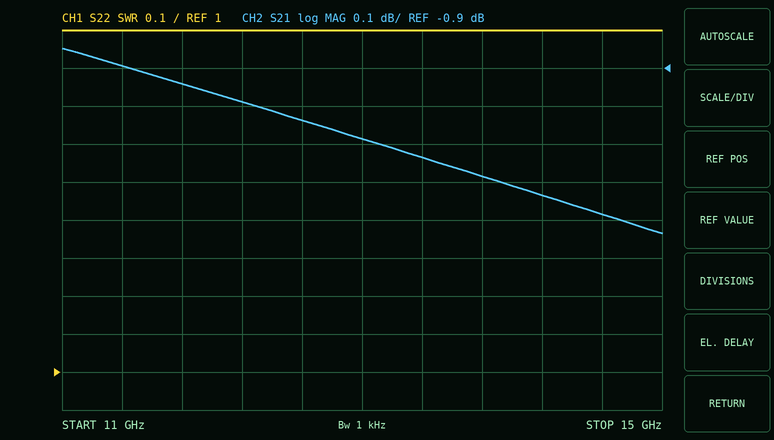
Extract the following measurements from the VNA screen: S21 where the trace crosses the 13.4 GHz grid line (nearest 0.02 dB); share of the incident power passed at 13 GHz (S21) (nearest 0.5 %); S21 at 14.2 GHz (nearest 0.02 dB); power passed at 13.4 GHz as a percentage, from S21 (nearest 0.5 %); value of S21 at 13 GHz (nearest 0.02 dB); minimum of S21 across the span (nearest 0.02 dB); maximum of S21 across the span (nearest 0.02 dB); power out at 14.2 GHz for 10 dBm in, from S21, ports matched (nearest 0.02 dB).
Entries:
-1.14 dB
78.0 %
-1.24 dB
77.0 %
-1.08 dB
-1.34 dB
-0.84 dB
8.76 dBm
